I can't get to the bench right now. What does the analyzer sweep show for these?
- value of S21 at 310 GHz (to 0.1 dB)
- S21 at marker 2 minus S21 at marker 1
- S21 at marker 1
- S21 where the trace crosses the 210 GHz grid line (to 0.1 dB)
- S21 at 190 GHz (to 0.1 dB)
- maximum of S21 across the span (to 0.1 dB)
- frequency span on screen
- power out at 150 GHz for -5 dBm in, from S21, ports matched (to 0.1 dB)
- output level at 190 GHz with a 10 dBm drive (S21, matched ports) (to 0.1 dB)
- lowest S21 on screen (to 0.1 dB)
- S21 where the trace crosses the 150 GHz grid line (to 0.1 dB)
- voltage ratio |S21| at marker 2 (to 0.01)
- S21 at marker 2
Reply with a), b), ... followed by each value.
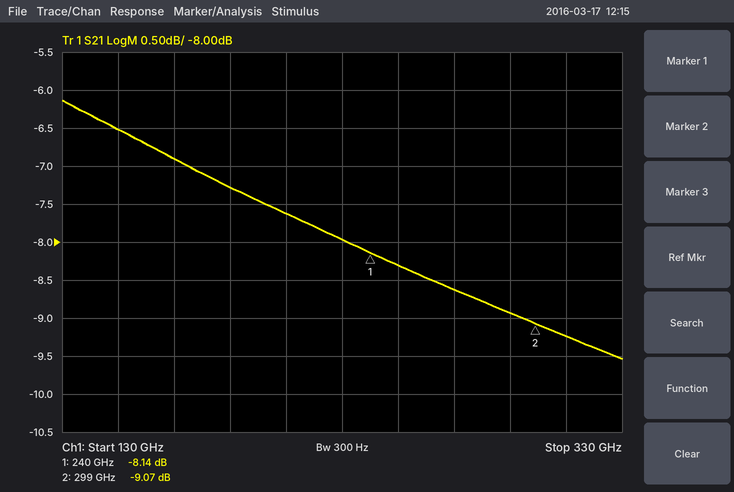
a) -9.2 dB
b) -0.93 dB
c) -8.14 dB
d) -7.6 dB
e) -7.3 dB
f) -6.1 dB
g) 200 GHz
h) -11.5 dBm
i) 2.7 dBm
j) -9.5 dB
k) -6.5 dB
l) 0.35
m) -9.07 dB
